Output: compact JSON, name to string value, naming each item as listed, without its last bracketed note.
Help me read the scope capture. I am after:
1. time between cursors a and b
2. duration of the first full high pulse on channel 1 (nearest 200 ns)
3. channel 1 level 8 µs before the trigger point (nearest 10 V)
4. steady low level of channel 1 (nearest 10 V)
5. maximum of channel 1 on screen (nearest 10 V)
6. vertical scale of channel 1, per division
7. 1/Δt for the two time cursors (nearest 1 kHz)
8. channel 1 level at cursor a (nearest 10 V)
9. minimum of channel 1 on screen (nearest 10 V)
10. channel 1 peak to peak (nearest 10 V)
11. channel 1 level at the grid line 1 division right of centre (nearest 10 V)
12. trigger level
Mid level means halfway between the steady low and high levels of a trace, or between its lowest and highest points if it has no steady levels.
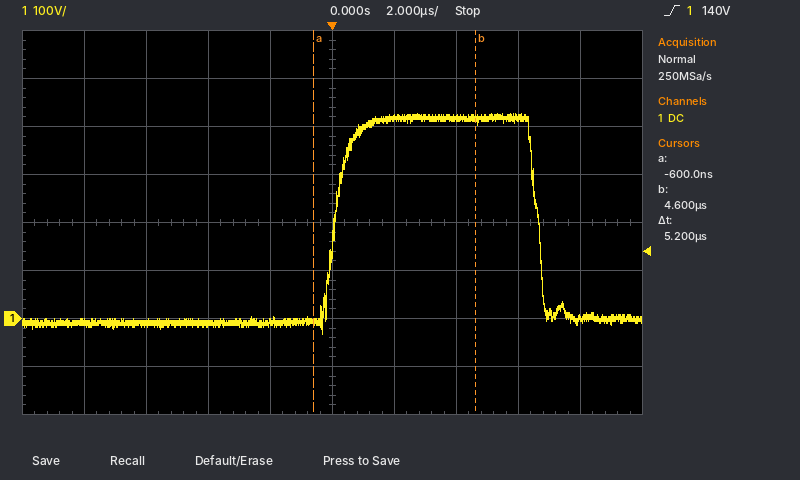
{"time between cursors a and b": "5.2 µs", "duration of the first full high pulse on channel 1": "6.6 µs", "channel 1 level 8 µs before the trigger point": "-10 V", "steady low level of channel 1": "-10 V", "maximum of channel 1 on screen": "430 V", "vertical scale of channel 1, per division": "100 V", "1/Δt for the two time cursors": "192 kHz", "channel 1 level at cursor a": "-10 V", "minimum of channel 1 on screen": "-30 V", "channel 1 peak to peak": "460 V", "channel 1 level at the grid line 1 division right of centre": "420 V", "trigger level": "140 V"}
